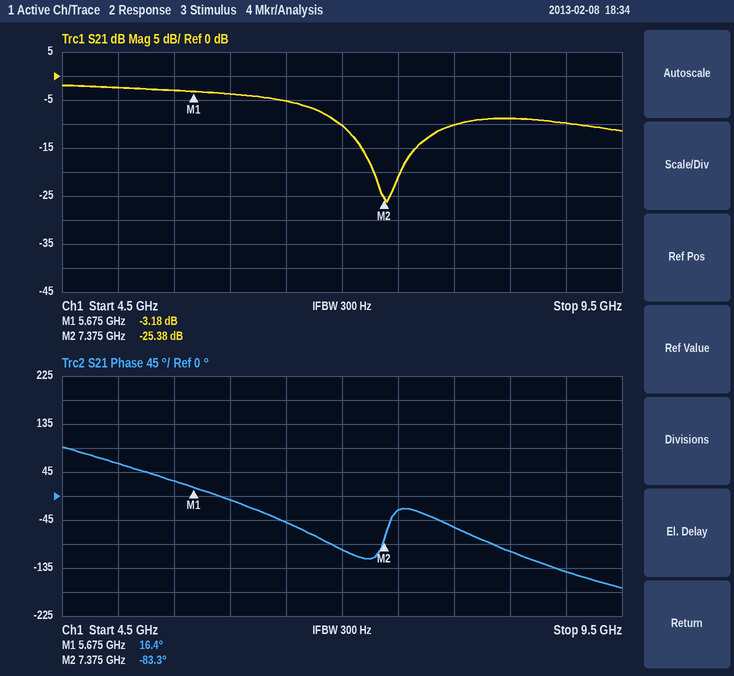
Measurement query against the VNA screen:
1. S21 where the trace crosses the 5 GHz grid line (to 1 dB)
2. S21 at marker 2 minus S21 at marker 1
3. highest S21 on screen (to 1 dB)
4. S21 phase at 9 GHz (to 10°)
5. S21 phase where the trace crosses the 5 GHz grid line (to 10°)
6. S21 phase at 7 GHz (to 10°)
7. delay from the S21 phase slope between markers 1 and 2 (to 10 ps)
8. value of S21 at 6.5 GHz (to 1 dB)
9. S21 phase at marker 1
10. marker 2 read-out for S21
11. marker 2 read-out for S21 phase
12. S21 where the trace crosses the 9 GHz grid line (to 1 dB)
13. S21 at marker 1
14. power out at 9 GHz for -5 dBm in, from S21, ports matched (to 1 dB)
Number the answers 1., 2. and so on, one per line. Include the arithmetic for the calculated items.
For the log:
1. -2 dB
2. -25.38 − (-3.18) = -22.20 dB
3. -2 dB
4. -140°
5. 60°
6. -100°
7. −(-83.3° − (16.4°))/(360° × 1.7 GHz) ≈ 163 ps, so 160 ps to the nearest 10 ps
8. -5 dB
9. 16.4°
10. -25.38 dB
11. -83.3°
12. -10 dB
13. -3.18 dB
14. -5 dBm + (-10 dB) = -15 dBm
